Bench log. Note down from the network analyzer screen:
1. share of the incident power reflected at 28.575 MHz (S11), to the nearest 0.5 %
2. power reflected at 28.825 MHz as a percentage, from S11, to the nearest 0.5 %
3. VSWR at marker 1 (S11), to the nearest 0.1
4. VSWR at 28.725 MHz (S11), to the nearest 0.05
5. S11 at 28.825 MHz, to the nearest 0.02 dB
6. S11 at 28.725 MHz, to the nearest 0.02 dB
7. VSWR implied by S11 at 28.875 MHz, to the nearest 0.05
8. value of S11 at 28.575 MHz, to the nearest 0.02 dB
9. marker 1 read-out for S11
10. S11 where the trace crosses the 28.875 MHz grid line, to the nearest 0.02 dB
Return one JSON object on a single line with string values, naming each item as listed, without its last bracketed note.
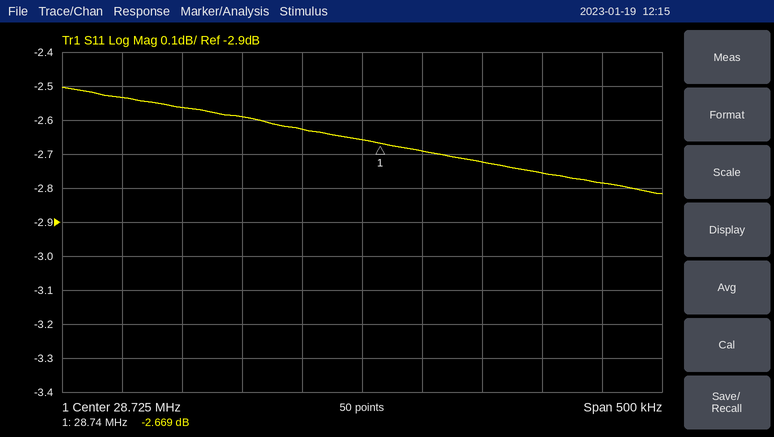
{"share of the incident power reflected at 28.575 MHz (S11), to the nearest 0.5 %": "55.5 %", "power reflected at 28.825 MHz as a percentage, from S11, to the nearest 0.5 %": "53.5 %", "VSWR at marker 1 (S11), to the nearest 0.1": "6.6", "VSWR at 28.725 MHz (S11), to the nearest 0.05": "6.60", "S11 at 28.825 MHz, to the nearest 0.02 dB": "-2.72 dB", "S11 at 28.725 MHz, to the nearest 0.02 dB": "-2.66 dB", "VSWR implied by S11 at 28.875 MHz, to the nearest 0.05": "6.35", "value of S11 at 28.575 MHz, to the nearest 0.02 dB": "-2.56 dB", "marker 1 read-out for S11": "-2.669 dB", "S11 where the trace crosses the 28.875 MHz grid line, to the nearest 0.02 dB": "-2.76 dB"}
